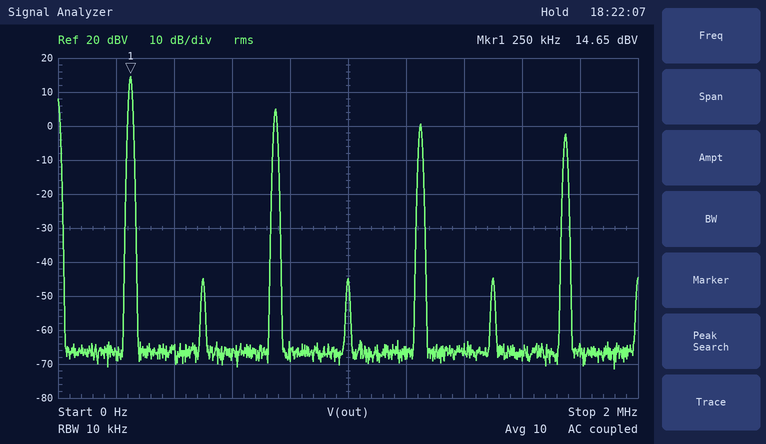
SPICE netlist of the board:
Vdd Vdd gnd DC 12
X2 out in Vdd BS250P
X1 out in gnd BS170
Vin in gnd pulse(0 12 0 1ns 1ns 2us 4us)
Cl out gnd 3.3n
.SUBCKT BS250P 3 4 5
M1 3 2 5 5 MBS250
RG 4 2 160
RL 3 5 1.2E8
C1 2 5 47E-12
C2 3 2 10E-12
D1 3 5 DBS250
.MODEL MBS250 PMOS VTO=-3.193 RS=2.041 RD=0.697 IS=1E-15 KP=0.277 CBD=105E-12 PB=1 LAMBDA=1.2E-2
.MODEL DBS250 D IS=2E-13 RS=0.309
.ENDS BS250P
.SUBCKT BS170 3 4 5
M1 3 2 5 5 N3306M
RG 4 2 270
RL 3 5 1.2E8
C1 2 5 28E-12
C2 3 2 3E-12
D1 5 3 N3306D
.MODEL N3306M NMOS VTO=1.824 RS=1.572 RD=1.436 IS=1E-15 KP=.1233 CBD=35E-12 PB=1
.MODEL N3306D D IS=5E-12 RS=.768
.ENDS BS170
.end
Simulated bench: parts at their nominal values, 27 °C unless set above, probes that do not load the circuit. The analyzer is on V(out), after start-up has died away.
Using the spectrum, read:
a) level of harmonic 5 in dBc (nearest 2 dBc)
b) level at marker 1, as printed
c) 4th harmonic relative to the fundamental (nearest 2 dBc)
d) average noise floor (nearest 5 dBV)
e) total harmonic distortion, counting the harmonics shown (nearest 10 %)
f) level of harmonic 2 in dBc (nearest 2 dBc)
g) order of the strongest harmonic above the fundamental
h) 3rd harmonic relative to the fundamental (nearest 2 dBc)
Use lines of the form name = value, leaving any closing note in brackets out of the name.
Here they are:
level of harmonic 5 in dBc = -14 dBc
level at marker 1, as printed = 14.65 dBV
4th harmonic relative to the fundamental = -60 dBc
average noise floor = -65 dBV
total harmonic distortion, counting the harmonics shown = 40 %
level of harmonic 2 in dBc = -60 dBc
order of the strongest harmonic above the fundamental = 3
3rd harmonic relative to the fundamental = -10 dBc
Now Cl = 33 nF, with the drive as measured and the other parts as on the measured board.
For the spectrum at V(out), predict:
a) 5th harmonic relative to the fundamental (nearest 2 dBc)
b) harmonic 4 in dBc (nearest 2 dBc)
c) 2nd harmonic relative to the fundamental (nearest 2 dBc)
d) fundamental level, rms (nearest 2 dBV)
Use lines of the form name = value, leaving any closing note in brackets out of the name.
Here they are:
5th harmonic relative to the fundamental = -16 dBc
harmonic 4 in dBc = -42 dBc
2nd harmonic relative to the fundamental = -40 dBc
fundamental level, rms = 14 dBV
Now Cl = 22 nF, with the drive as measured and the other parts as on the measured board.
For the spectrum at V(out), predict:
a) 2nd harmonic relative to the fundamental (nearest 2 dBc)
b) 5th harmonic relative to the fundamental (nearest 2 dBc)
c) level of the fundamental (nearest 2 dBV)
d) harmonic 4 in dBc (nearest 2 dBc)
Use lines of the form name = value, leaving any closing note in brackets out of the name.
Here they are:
2nd harmonic relative to the fundamental = -44 dBc
5th harmonic relative to the fundamental = -16 dBc
level of the fundamental = 14 dBV
harmonic 4 in dBc = -46 dBc
